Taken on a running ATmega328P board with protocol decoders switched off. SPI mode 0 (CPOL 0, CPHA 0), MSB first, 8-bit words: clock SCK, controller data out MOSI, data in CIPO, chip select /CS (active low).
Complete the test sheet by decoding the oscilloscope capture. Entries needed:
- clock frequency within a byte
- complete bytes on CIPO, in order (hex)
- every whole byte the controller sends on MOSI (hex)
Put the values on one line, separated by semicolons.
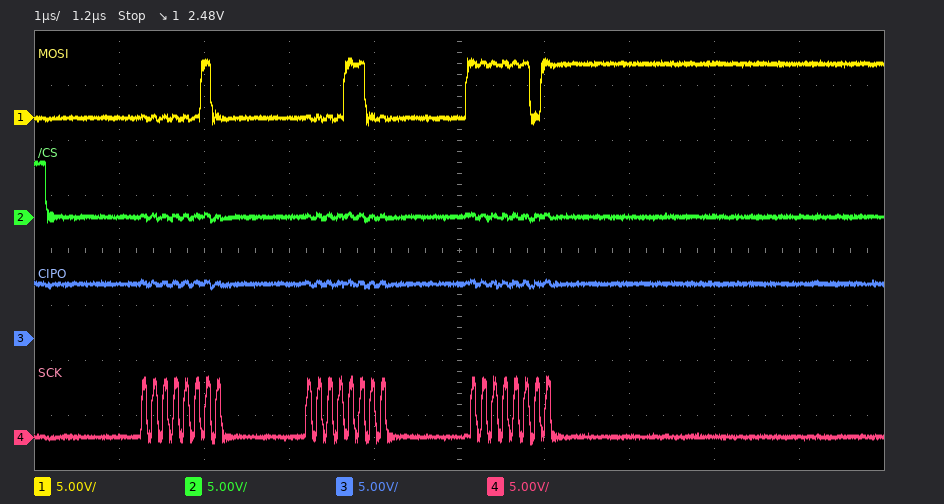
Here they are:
8 MHz; FF FF FF; 02 0C FD
